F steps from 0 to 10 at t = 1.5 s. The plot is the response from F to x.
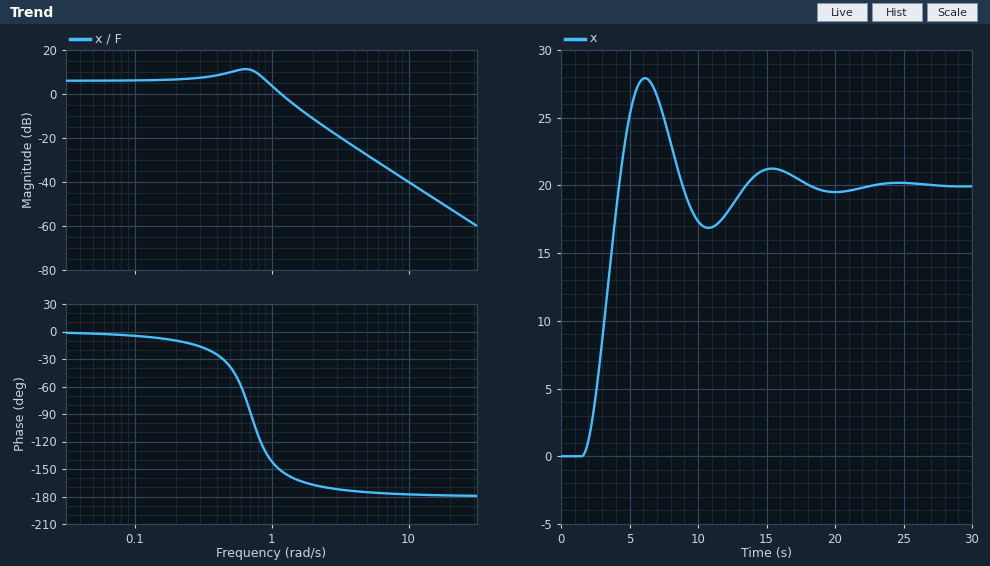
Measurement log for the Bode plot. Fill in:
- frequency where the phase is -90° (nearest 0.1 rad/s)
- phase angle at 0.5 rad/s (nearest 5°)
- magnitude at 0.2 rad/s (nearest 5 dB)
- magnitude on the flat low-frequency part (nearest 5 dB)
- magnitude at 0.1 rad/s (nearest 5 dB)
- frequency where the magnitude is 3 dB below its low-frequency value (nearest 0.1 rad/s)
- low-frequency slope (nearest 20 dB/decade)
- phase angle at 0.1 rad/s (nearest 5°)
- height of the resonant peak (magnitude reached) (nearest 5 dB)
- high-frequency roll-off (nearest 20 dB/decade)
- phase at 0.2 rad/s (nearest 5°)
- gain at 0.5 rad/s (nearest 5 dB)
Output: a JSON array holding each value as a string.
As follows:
["0.7 rad/s", "-40°", "5 dB", "5 dB", "5 dB", "1.0 rad/s", "0 dB/decade", "-5°", "10 dB", "-40 dB/decade", "-10°", "10 dB"]
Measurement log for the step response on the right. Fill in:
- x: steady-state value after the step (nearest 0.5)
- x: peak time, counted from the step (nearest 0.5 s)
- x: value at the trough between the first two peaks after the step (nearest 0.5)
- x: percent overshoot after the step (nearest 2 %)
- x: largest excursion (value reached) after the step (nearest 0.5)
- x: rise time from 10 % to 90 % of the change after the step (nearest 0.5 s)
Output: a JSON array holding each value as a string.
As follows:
["20.0", "4.5 s", "17.0", "40 %", "28.0", "2.0 s"]
